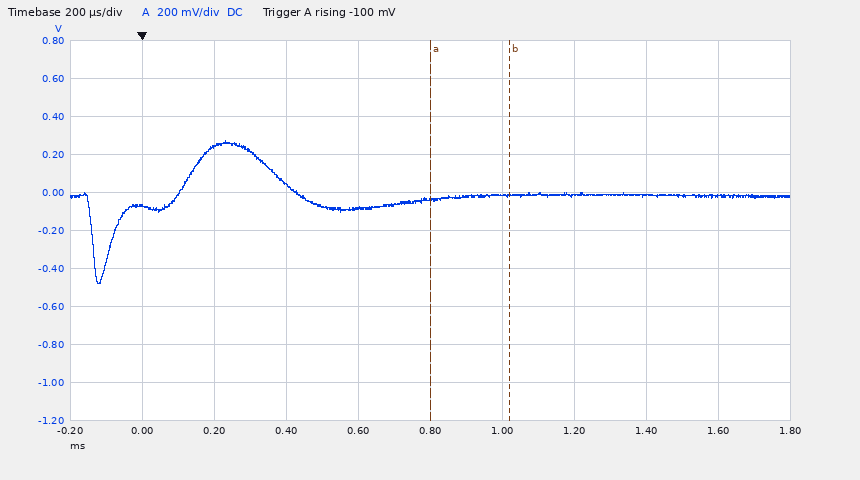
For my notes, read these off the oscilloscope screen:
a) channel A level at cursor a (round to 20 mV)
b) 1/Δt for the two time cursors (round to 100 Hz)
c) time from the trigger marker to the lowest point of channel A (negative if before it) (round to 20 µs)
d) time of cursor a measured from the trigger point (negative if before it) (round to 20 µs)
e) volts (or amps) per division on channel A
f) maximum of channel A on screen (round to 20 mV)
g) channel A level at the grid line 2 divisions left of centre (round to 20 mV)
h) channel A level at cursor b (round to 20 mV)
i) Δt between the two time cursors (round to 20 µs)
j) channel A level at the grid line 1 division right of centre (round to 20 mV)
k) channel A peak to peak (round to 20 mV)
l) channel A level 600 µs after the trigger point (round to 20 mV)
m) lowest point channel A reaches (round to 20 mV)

-40 mV
4.5 kHz
-120 µs
+800 µs
200 mV
280 mV
40 mV
-20 mV
220 µs
-20 mV
760 mV
-80 mV
-480 mV
